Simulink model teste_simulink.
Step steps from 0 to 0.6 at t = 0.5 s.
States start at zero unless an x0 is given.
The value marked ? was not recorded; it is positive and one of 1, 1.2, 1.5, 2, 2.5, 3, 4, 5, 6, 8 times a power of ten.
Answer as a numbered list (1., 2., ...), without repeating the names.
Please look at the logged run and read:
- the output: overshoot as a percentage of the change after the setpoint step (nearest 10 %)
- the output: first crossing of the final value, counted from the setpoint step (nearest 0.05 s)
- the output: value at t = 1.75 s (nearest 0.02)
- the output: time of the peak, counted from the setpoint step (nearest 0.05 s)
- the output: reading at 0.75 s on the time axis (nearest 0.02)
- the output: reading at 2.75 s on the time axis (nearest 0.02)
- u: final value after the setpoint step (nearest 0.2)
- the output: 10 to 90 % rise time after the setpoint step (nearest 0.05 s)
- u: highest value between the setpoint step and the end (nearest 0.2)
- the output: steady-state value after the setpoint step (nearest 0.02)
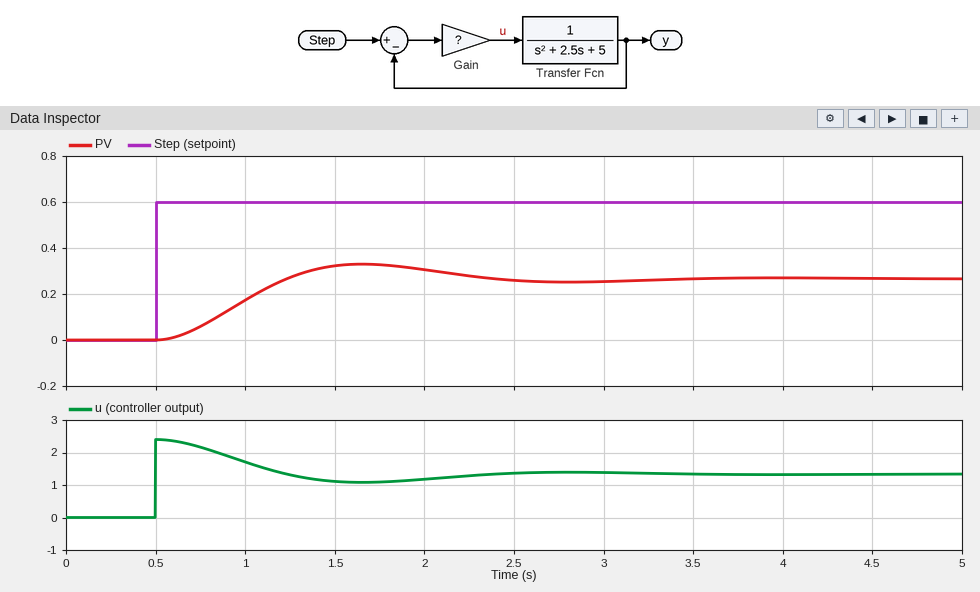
1. 20 %
2. 0.75 s
3. 0.32
4. 1.15 s
5. 0.06
6. 0.26
7. 1.4
8. 0.50 s
9. 2.4
10. 0.26
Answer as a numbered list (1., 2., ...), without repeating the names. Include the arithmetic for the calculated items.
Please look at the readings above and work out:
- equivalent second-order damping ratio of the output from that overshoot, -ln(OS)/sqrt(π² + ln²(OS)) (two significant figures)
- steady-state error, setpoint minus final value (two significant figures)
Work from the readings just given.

1. ln(0.2) = -1.609; 1.609 / sqrt(9.870 + 2.590) = 0.46
2. 0.6 - 0.26 = 0.34
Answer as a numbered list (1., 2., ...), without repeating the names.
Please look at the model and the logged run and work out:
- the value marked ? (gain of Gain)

1. 4
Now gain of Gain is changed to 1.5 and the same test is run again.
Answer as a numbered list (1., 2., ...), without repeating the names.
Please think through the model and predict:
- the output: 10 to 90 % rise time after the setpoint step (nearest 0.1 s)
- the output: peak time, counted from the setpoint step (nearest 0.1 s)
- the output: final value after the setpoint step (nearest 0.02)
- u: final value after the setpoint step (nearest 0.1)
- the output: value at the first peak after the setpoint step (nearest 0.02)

1. 0.6 s
2. 1.4 s
3. 0.14
4. 0.7
5. 0.16
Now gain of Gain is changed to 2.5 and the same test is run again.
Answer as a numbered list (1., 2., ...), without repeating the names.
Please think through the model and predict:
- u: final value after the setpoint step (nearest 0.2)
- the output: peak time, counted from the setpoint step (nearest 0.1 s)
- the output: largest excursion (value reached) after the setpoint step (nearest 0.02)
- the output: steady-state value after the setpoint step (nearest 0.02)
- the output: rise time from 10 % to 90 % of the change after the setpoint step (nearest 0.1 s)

1. 1.0
2. 1.3 s
3. 0.24
4. 0.20
5. 0.6 s
